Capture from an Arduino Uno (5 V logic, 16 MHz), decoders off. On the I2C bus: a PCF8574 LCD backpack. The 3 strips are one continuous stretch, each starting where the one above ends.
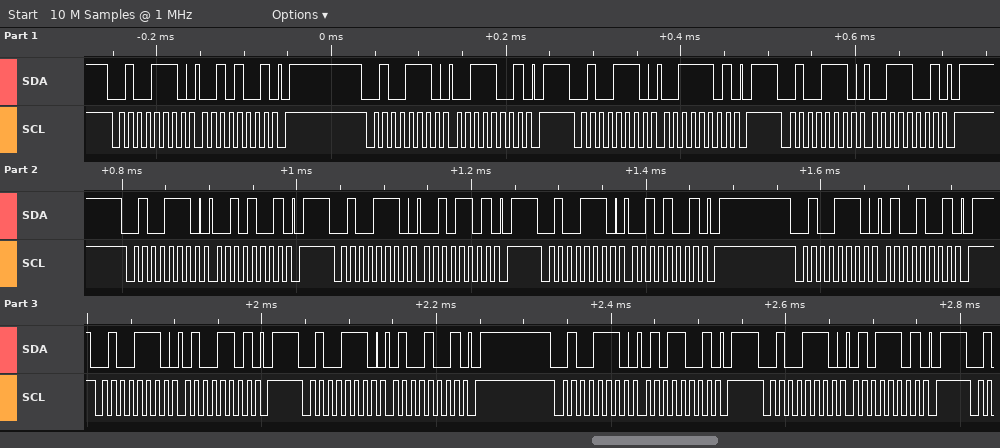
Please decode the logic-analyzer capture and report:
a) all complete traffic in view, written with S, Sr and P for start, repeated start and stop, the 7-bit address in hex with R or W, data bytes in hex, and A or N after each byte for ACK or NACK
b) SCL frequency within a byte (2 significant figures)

S 27W A 29 A P S 27W A 39 A P S 27W A 3D A P S 27W A 39 A P S 27W A 29 A P S 27W A 2D A P S 27W A 29 A P S 27W A 49 A P S 27W A 4D A P S 27W A 49 A P S 27W A 59 A P S 27W A 5D A P
100 kHz
